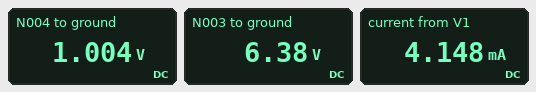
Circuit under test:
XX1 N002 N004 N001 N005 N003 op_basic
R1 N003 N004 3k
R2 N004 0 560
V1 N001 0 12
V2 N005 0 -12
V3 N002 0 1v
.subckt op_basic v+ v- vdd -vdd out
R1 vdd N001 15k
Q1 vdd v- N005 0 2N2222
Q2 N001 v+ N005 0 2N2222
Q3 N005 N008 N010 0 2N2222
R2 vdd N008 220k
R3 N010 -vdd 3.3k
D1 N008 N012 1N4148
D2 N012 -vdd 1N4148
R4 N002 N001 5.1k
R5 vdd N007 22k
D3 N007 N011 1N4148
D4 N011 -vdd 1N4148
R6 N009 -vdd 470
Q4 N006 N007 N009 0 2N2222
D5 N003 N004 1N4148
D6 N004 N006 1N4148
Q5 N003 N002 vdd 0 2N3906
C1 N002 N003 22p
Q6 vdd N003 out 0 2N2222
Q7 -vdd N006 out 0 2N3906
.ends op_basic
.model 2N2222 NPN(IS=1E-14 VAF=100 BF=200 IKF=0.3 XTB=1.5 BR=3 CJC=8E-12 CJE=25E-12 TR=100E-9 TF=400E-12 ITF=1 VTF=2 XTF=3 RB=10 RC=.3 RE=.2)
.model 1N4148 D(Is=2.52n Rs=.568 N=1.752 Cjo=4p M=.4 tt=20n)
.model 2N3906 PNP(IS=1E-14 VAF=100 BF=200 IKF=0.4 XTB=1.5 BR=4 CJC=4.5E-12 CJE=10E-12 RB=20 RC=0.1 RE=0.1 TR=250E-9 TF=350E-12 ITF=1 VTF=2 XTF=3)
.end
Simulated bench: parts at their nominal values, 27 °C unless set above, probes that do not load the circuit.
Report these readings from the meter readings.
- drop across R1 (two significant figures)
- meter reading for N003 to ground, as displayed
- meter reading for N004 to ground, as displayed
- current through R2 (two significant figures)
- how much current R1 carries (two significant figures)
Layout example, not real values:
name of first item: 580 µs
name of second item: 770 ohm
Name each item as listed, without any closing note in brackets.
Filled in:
drop across R1: 5.4 V
meter reading for N003 to ground, as displayed: 6.38 V
meter reading for N004 to ground, as displayed: 1.004 V
current through R2: 1.8 mA
how much current R1 carries: 1.8 mA
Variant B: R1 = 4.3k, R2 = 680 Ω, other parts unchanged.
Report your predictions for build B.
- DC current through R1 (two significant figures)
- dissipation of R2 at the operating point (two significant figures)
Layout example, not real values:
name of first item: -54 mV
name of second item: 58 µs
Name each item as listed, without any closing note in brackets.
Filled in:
DC current through R1: 1.5 mA
dissipation of R2 at the operating point: 1.5 mW
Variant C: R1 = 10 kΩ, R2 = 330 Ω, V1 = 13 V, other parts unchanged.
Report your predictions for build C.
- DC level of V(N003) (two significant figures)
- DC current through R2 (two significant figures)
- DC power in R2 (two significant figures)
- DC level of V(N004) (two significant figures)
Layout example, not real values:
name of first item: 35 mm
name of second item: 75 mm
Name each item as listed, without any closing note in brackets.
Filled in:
DC level of V(N003): 12 V
DC current through R2: 1.2 mA
DC power in R2: 470 µW
DC level of V(N004): 390 mV
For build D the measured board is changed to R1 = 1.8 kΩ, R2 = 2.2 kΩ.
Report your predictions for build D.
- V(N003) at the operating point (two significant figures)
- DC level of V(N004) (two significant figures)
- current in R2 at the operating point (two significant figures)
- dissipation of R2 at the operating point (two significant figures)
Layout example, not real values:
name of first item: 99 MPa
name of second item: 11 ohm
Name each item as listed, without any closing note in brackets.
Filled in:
V(N003) at the operating point: 1.8 V
DC level of V(N004): 1.0 V
current in R2 at the operating point: 460 µA
dissipation of R2 at the operating point: 460 µW
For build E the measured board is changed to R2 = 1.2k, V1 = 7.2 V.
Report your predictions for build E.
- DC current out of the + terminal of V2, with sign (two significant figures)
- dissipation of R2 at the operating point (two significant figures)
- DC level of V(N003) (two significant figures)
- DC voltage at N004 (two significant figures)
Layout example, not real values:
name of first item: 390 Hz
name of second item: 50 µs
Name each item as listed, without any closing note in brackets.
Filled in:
DC current out of the + terminal of V2, with sign: -2.1 mA
dissipation of R2 at the operating point: 840 µW
DC level of V(N003): 3.5 V
DC voltage at N004: 1.0 V
